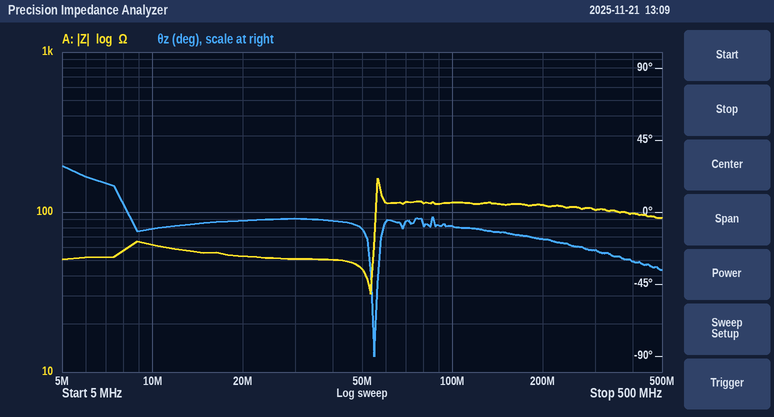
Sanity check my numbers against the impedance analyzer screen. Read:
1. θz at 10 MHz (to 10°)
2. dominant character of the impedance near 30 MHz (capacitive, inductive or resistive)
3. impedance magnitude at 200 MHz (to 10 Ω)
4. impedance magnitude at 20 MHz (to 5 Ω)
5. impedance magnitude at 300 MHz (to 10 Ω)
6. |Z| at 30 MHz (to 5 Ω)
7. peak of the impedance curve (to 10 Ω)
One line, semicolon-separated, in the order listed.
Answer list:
-10°; resistive; 110 Ω; 55 Ω; 100 Ω; 50 Ω; 160 Ω
